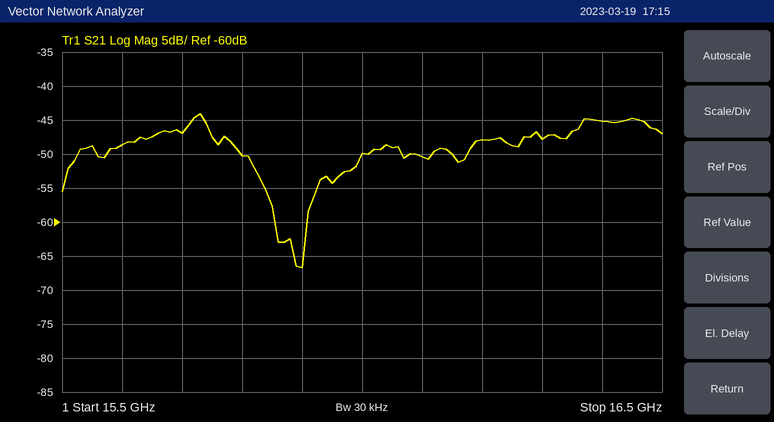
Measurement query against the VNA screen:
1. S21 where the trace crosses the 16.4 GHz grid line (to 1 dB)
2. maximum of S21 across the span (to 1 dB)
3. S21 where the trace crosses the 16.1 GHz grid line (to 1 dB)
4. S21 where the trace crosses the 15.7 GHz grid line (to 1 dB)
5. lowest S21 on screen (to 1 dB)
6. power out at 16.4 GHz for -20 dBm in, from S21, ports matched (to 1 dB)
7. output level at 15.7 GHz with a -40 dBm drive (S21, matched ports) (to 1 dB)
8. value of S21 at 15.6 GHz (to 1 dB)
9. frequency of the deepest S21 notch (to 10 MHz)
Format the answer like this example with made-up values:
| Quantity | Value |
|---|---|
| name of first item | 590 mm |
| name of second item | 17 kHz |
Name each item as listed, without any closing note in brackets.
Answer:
| Quantity | Value |
|---|---|
| S21 where the trace crosses the 16.4 GHz grid line | -45 dB |
| maximum of S21 across the span | -44 dB |
| S21 where the trace crosses the 16.1 GHz grid line | -50 dB |
| S21 where the trace crosses the 15.7 GHz grid line | -47 dB |
| lowest S21 on screen | -67 dB |
| power out at 16.4 GHz for -20 dBm in, from S21, ports matched | -65 dBm |
| output level at 15.7 GHz with a -40 dBm drive (S21, matched ports) | -87 dBm |
| value of S21 at 15.6 GHz | -49 dB |
| frequency of the deepest S21 notch | 15.90 GHz |
